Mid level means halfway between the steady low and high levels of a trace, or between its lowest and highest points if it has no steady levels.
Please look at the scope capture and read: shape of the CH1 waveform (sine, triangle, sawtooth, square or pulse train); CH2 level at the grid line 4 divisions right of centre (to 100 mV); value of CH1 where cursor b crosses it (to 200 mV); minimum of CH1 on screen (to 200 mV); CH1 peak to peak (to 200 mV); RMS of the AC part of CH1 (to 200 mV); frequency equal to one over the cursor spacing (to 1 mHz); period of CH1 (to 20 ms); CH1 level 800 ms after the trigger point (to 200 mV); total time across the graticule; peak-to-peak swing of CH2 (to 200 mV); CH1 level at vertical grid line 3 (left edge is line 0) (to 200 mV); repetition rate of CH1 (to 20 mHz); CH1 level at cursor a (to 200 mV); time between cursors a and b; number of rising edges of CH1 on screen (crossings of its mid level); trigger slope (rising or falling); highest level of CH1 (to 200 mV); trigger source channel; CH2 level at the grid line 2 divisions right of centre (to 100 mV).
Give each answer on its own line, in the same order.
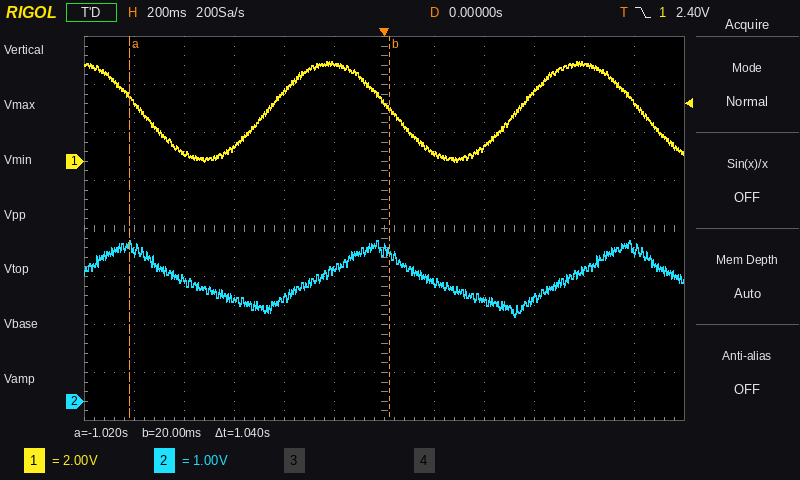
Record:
sine
2.7 V
2.2 V
0.0 V
4.2 V
1.4 V
962 mHz
1.00 s
4.0 V
2.4 s
1.6 V
600 mV
1.00 Hz
2.8 V
1.04 s
2
falling
4.2 V
CH1
2.1 V
